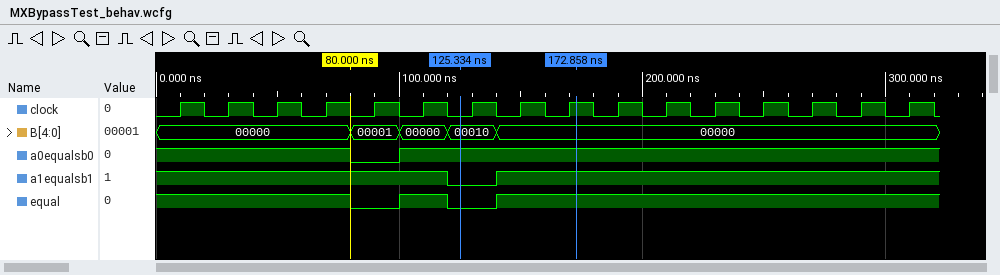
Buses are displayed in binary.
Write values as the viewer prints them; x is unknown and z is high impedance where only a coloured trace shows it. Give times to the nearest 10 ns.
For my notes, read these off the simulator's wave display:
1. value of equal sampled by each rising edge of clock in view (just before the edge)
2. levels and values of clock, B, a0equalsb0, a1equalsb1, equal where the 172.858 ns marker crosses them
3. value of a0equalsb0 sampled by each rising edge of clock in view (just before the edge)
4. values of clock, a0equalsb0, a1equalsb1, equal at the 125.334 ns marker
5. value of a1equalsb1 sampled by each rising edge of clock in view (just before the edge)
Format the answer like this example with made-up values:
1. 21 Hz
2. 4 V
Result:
1. 1 1 1 1 0 1 0 1 1 1 1 1 1 1 1 1
2. clock=1, B=00000, a0equalsb0=1, a1equalsb1=1, equal=1
3. 1 1 1 1 0 1 1 1 1 1 1 1 1 1 1 1
4. clock=0, a0equalsb0=1, a1equalsb1=0, equal=0
5. 1 1 1 1 1 1 0 1 1 1 1 1 1 1 1 1
